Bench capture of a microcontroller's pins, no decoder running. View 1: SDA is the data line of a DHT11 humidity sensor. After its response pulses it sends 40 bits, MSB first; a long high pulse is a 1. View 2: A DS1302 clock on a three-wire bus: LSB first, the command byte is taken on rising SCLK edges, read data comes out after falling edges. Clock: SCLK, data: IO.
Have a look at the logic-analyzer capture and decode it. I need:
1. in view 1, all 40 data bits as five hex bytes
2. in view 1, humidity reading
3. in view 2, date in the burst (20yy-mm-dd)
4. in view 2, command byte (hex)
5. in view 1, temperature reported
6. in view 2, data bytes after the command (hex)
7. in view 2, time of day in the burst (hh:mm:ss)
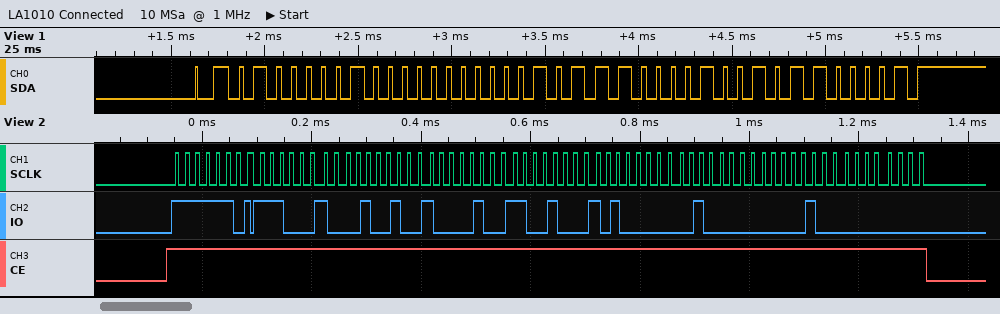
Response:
41 00 17 09 61
65 %
2020-05-13
0xBF
23.9 °C
47 24 21 13 05 04 20 00
21:24:47
